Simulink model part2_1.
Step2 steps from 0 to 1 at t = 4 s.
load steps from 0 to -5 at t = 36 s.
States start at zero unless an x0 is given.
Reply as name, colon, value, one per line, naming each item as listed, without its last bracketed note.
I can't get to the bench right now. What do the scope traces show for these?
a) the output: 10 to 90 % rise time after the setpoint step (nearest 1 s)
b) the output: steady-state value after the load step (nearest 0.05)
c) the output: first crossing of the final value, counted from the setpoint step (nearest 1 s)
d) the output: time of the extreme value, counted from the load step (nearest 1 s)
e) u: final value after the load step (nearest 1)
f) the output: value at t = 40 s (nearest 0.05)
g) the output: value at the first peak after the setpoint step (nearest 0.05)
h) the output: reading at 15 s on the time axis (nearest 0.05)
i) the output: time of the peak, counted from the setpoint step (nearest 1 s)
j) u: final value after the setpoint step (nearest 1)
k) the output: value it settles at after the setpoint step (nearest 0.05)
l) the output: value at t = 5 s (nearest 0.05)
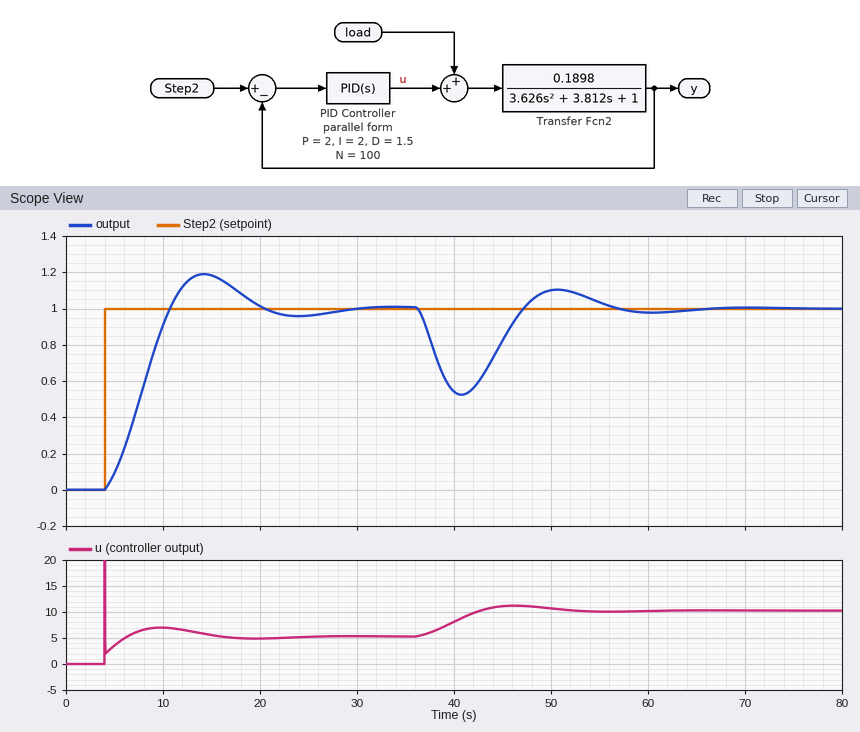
the output: 10 to 90 % rise time after the setpoint step: 5 s
the output: steady-state value after the load step: 1.00
the output: first crossing of the final value, counted from the setpoint step: 7 s
the output: time of the extreme value, counted from the load step: 5 s
u: final value after the load step: 10
the output: value at t = 40 s: 0.55
the output: value at the first peak after the setpoint step: 1.20
the output: reading at 15 s on the time axis: 1.20
the output: time of the peak, counted from the setpoint step: 10 s
u: final value after the setpoint step: 5
the output: value it settles at after the setpoint step: 1.00
the output: value at t = 5 s: 0.10
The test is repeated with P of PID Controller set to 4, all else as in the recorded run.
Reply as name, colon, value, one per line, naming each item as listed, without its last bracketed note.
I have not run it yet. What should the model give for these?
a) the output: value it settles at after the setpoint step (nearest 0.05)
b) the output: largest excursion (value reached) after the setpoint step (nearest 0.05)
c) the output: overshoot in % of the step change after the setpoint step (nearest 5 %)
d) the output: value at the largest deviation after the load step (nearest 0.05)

the output: value it settles at after the setpoint step: 1.00
the output: largest excursion (value reached) after the setpoint step: 1.10
the output: overshoot in % of the step change after the setpoint step: 10 %
the output: value at the largest deviation after the load step: 0.60
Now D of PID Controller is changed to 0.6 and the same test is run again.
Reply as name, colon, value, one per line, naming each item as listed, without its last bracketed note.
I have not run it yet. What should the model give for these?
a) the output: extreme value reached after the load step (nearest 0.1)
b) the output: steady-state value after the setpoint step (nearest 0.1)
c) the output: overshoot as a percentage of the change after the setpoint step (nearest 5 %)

the output: extreme value reached after the load step: 0.5
the output: steady-state value after the setpoint step: 1.0
the output: overshoot as a percentage of the change after the setpoint step: 20 %
